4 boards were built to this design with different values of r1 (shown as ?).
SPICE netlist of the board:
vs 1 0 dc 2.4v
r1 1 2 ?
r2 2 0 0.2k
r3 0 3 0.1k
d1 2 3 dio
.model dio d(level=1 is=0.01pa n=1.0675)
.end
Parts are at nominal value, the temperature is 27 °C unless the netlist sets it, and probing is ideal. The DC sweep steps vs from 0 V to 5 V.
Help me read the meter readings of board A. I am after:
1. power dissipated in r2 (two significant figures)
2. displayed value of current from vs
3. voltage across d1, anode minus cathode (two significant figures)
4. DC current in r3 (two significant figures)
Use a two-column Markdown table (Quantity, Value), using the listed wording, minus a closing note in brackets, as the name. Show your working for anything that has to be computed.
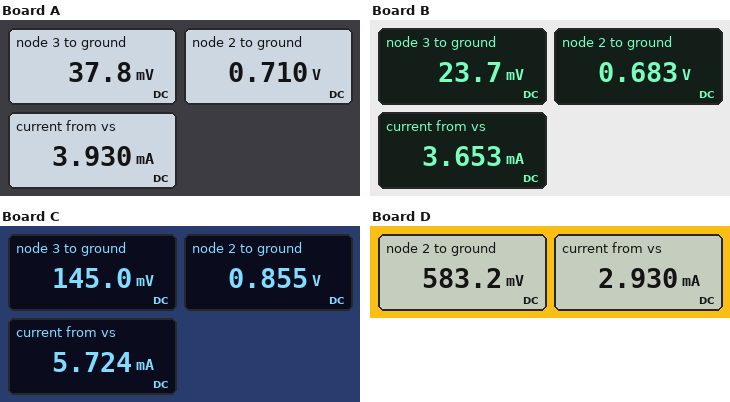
| Quantity | Value |
|---|---|
| power dissipated in r2 | (710 mV)^2 / 200 Ω = 2.5 mW |
| displayed value of current from vs | 3.930 mA |
| voltage across d1, anode minus cathode | 710 mV - 37.8 mV = 670 mV |
| DC current in r3 | (37.8 mV) / 100 Ω = 380 µA |
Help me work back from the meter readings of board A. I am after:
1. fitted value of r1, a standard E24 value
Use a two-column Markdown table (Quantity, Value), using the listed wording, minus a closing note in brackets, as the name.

| Quantity | Value |
|---|---|
| fitted value of r1, a standard E24 value | 430 Ω |
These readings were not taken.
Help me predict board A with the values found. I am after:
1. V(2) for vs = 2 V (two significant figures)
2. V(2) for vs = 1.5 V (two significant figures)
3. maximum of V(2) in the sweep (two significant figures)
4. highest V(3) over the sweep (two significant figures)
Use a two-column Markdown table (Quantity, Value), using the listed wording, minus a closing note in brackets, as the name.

| Quantity | Value |
|---|---|
| V(2) for vs = 2 V | 630 mV |
| V(2) for vs = 1.5 V | 480 mV |
| maximum of V(2) in the sweep | 1.1 V |
| highest V(3) over the sweep | 360 mV |
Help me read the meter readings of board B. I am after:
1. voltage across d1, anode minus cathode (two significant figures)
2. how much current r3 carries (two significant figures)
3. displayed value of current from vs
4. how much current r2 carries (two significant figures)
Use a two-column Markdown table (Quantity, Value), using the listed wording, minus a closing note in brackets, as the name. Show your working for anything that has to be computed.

| Quantity | Value |
|---|---|
| voltage across d1, anode minus cathode | 683 mV - 23.7 mV = 660 mV |
| how much current r3 carries | (23.7 mV) / 100 Ω = 240 µA |
| displayed value of current from vs | 3.653 mA |
| how much current r2 carries | (683 mV) / 200 Ω = 3.4 mA |
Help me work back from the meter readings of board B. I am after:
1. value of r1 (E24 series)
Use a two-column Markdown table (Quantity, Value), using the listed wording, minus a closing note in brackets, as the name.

| Quantity | Value |
|---|---|
| value of r1 | 470 Ω |
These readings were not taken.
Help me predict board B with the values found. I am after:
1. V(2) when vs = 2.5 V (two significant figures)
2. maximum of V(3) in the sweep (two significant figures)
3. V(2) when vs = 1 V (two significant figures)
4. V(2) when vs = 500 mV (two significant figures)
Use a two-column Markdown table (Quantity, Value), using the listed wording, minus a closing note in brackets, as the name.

| Quantity | Value |
|---|---|
| V(2) when vs = 2.5 V | 700 mV |
| maximum of V(3) in the sweep | 320 mV |
| V(2) when vs = 1 V | 300 mV |
| V(2) when vs = 500 mV | 150 mV |
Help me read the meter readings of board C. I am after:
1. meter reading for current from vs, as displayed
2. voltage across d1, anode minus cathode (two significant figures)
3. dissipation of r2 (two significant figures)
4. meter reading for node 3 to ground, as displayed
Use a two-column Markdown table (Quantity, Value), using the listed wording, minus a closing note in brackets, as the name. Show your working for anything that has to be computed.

| Quantity | Value |
|---|---|
| meter reading for current from vs, as displayed | 5.724 mA |
| voltage across d1, anode minus cathode | 855 mV - 145 mV = 710 mV |
| dissipation of r2 | (855 mV)^2 / 200 Ω = 3.7 mW |
| meter reading for node 3 to ground, as displayed | 145.0 mV |
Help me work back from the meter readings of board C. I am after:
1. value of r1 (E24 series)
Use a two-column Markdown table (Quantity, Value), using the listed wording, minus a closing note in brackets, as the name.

| Quantity | Value |
|---|---|
| value of r1 | 270 Ω |
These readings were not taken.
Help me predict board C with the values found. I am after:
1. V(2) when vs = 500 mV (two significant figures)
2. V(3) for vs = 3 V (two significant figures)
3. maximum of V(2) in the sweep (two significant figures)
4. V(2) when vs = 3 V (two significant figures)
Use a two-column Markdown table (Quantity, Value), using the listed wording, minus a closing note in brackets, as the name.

| Quantity | Value |
|---|---|
| V(2) when vs = 500 mV | 210 mV |
| V(3) for vs = 3 V | 260 mV |
| maximum of V(2) in the sweep | 1.4 V |
| V(2) when vs = 3 V | 980 mV |
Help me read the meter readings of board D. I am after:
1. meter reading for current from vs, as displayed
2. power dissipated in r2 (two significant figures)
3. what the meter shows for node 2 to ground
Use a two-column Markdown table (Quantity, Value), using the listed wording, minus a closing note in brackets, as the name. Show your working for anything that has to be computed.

| Quantity | Value |
|---|---|
| meter reading for current from vs, as displayed | 2.930 mA |
| power dissipated in r2 | (583.2 mV)^2 / 200 Ω = 1.7 mW |
| what the meter shows for node 2 to ground | 583.2 mV |
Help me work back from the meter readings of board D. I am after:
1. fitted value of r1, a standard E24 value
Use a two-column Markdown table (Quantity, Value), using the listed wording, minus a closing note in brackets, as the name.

| Quantity | Value |
|---|---|
| fitted value of r1, a standard E24 value | 620 Ω |
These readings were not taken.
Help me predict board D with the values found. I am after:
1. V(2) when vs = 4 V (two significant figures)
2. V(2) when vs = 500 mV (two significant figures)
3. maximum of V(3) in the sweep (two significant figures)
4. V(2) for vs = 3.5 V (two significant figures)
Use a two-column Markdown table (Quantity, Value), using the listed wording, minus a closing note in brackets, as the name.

| Quantity | Value |
|---|---|
| V(2) when vs = 4 V | 810 mV |
| V(2) when vs = 500 mV | 120 mV |
| maximum of V(3) in the sweep | 200 mV |
| V(2) for vs = 3.5 V | 750 mV |
